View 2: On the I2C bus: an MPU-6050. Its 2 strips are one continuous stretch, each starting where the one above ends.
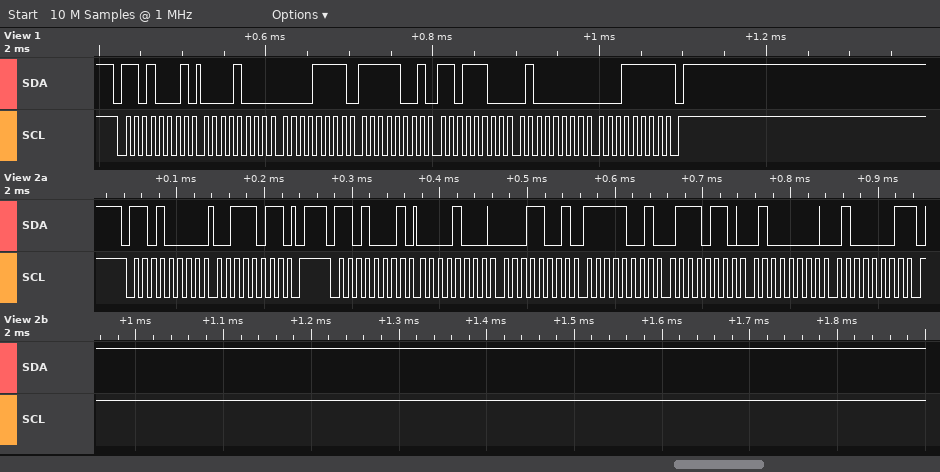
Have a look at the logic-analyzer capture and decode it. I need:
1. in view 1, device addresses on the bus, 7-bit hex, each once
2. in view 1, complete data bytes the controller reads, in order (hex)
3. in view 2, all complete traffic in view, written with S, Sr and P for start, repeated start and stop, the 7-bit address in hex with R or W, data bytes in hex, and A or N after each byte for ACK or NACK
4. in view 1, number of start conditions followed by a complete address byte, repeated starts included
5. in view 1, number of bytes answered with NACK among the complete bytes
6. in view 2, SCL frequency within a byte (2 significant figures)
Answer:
0x68
08 0F F9 DC 40 1F
S 68W A 3B A P S 68R A 08 A 19 A F9 A 76 A 40 A 41 N P
1
1
100 kHz
